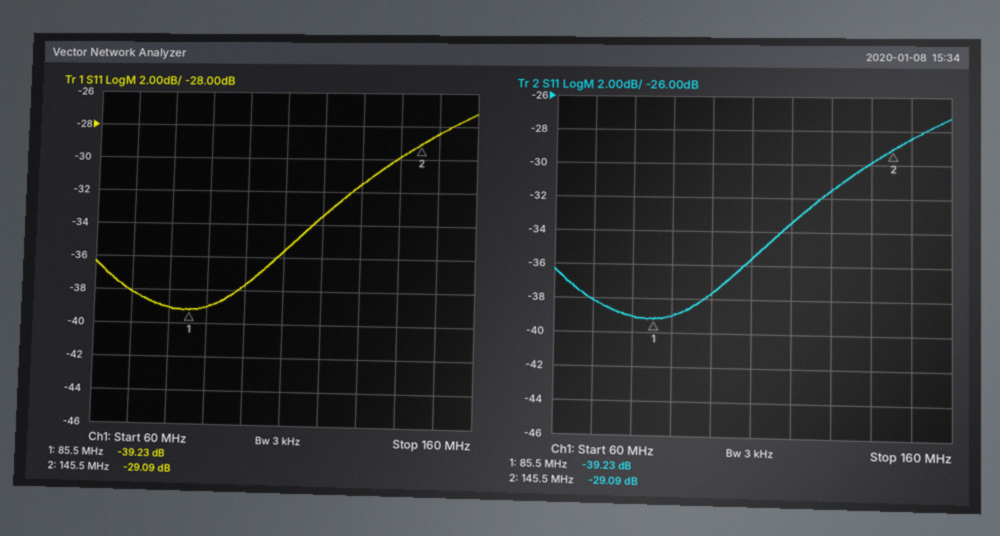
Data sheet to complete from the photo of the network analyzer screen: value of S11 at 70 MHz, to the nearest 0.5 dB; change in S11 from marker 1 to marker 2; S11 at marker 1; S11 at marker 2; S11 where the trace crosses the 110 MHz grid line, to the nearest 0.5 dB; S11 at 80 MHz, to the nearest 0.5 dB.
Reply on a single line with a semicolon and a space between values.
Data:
-38.0 dB; 10.14 dB; -39.23 dB; -29.09 dB; -35.5 dB; -39.0 dB
